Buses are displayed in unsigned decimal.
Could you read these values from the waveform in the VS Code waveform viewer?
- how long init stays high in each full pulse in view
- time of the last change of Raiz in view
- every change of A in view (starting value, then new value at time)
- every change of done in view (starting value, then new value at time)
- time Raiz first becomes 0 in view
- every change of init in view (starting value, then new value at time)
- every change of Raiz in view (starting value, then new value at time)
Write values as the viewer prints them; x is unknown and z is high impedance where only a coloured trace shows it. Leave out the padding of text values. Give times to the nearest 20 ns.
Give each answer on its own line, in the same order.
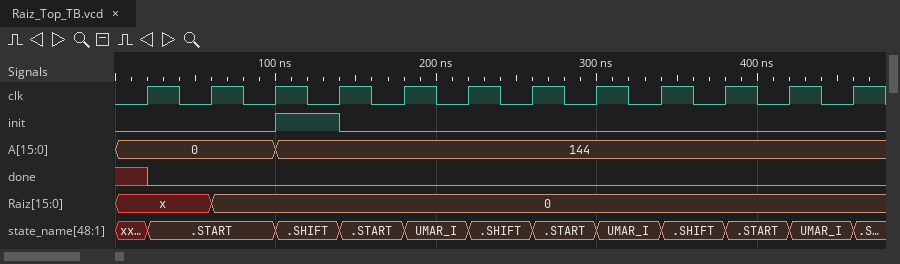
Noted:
40 ns
60 ns
0, 144 at 100 ns
x, 0 at 20 ns
60 ns
0, 1 at 100 ns, 0 at 140 ns
x, 0 at 60 ns
